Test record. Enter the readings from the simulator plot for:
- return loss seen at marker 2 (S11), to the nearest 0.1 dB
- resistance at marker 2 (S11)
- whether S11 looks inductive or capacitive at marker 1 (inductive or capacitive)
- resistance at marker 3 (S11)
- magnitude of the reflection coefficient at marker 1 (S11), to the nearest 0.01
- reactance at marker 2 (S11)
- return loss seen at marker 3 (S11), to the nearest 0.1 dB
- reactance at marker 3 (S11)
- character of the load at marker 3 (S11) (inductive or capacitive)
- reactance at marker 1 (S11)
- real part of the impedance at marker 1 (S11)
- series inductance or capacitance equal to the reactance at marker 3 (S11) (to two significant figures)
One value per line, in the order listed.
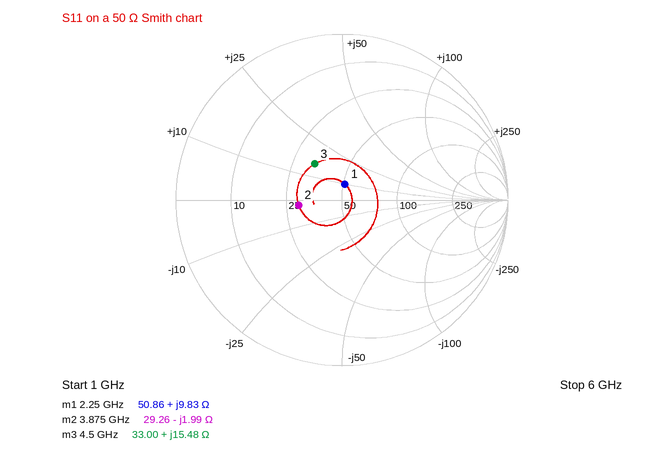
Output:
11.6 dB
29.26 Ω
inductive
33.00 Ω
0.10
-1.99 Ω
11.3 dB
+15.48 Ω
inductive
+9.83 Ω
50.86 Ω
550 pH
